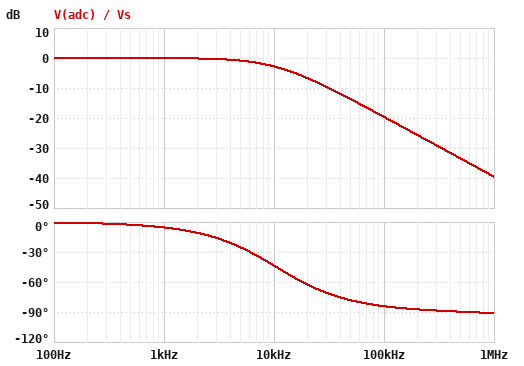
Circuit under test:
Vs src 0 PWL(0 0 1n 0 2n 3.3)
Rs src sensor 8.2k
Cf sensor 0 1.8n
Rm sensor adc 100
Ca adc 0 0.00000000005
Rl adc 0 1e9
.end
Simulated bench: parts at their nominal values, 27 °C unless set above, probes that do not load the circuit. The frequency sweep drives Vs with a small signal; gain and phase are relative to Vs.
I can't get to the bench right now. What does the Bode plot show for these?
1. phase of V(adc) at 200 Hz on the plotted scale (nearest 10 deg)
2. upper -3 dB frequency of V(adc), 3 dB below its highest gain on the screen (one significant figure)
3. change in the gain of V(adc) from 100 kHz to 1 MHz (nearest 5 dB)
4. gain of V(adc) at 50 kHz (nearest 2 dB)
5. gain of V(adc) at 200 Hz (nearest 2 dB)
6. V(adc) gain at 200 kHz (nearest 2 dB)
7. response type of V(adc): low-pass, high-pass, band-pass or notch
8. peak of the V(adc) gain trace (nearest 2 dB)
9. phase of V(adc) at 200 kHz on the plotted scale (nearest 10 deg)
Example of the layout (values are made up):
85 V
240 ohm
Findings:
0 deg
10 kHz
-20 dB
-14 dB
0 dB
-26 dB
low-pass
0 dB
-90 deg
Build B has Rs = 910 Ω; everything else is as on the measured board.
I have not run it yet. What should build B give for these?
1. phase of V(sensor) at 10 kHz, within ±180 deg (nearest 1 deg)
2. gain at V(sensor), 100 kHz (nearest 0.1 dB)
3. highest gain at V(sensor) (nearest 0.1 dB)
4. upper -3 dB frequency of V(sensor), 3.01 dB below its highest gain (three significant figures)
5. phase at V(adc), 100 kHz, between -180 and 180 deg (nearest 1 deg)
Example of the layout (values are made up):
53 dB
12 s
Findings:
-6 deg
-3.3 dB
0 dB
94.5 kHz
-47 deg
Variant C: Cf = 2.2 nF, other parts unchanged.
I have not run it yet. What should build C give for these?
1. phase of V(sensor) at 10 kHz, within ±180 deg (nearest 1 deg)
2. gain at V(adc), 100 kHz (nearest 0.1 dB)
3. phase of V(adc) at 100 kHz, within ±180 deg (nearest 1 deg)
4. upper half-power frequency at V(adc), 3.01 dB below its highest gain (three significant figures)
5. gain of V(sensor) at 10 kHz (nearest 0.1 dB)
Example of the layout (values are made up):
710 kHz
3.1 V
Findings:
-49 deg
-21.3 dB
-85 deg
8.63 kHz
-3.7 dB
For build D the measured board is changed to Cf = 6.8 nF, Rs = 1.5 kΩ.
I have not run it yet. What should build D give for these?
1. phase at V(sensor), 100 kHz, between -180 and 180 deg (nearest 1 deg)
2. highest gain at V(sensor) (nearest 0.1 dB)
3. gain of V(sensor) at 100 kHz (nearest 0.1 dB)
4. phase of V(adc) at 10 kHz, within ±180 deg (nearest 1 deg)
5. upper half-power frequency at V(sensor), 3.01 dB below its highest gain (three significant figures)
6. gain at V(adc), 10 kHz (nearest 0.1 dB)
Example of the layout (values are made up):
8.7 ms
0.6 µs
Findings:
-81 deg
0 dB
-16.3 dB
-33 deg
15.5 kHz
-1.5 dB
